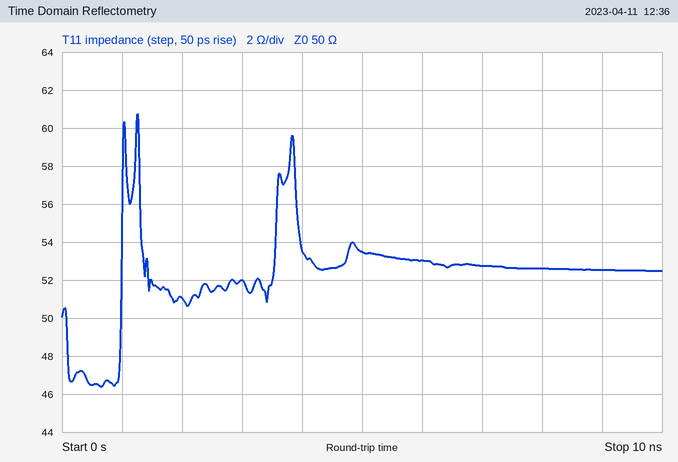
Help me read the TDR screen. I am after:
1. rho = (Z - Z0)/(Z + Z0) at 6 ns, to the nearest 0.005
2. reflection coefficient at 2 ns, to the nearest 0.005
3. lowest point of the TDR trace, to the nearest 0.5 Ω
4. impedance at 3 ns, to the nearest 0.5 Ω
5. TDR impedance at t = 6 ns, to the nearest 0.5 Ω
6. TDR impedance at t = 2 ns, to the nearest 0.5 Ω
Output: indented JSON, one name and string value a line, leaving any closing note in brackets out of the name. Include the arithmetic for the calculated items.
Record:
{
  "rho = (Z - Z0)/(Z + Z0) at 6 ns, to the nearest 0.005": "(53 − 50)/(53 + 50) ≈ +0.0291, so +0.030 to the nearest 0.005",
  "reflection coefficient at 2 ns, to the nearest 0.005": "(51 − 50)/(51 + 50) ≈ +0.010",
  "lowest point of the TDR trace, to the nearest 0.5 Ω": "46.5 Ω",
  "impedance at 3 ns, to the nearest 0.5 Ω": "52.0 Ω",
  "TDR impedance at t = 6 ns, to the nearest 0.5 Ω": "53.0 Ω",
  "TDR impedance at t = 2 ns, to the nearest 0.5 Ω": "51.0 Ω"
}
